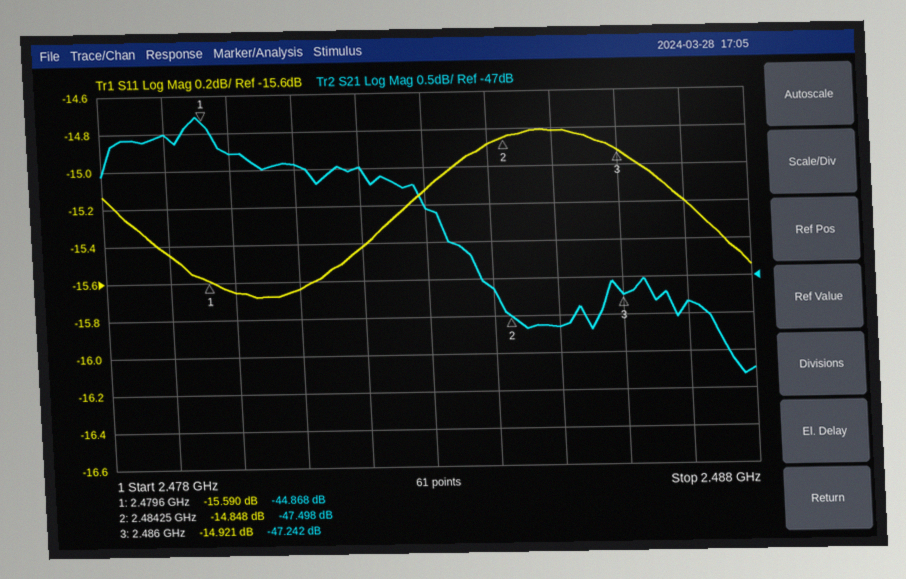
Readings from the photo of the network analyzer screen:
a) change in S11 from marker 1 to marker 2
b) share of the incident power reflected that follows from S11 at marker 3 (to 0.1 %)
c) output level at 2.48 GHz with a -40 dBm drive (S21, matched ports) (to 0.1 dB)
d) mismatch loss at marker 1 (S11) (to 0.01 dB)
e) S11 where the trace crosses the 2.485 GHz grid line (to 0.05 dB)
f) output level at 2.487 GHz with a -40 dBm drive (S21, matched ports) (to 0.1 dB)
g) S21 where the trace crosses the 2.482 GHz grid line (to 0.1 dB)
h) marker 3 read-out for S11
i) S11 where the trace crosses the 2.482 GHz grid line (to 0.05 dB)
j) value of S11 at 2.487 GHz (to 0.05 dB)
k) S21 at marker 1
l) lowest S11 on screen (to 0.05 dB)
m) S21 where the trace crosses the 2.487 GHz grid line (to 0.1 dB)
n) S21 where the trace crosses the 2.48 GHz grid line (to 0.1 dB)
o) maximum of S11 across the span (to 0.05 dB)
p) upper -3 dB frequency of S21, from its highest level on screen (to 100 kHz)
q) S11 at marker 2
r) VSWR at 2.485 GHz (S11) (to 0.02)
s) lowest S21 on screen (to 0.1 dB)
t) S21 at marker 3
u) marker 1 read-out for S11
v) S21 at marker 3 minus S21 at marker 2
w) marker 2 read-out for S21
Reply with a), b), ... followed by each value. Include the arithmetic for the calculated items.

a) -14.848 − (-15.59) = 0.742 dB
b) 10^(-14.921/10) ≈ 3.2 %
c) -40 dBm + (-45.3 dB) = -85.3 dBm
d) −10 log10(1 − 10^(-15.59/10)) ≈ 0.12 dB
e) -14.80 dB
f) -40 dBm + (-47.3 dB) = -87.3 dBm
g) -45.5 dB
h) -14.921 dB
i) -15.40 dB
j) -15.20 dB
k) -44.868 dB
l) -15.70 dB
m) -47.3 dB
n) -45.3 dB
o) -14.80 dB
p) 2.4875 GHz
q) -14.848 dB
r) |Γ| = 10^(-14.8/20) = 0.1820; VSWR = (1 + 0.1820)/(1 − 0.1820) ≈ 1.44
s) -48.3 dB
t) -47.242 dB
u) -15.590 dB
v) -47.242 − (-47.498) = 0.256 dB
w) -47.498 dB
